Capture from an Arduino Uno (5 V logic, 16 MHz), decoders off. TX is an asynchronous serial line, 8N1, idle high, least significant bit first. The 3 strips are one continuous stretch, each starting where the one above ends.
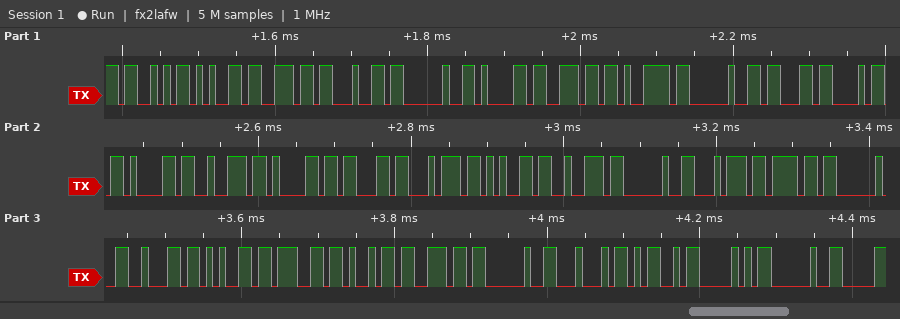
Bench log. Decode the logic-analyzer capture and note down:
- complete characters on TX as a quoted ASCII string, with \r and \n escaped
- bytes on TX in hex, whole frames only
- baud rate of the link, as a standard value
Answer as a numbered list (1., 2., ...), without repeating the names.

1. "Send any character to begin DMP "
2. 53 65 6E 64 20 61 6E 79 20 63 68 61 72 61 63 74 65 72 20 74 6F 20 62 65 67 69 6E 20 44 4D 50 20
3. 115200 baud
